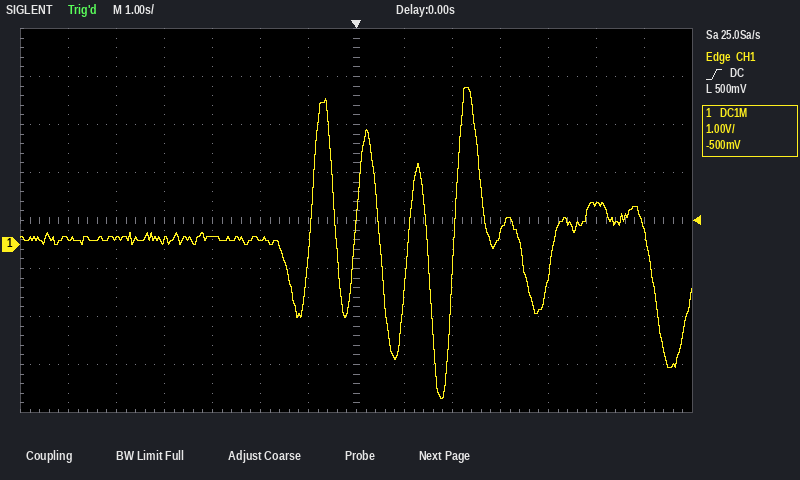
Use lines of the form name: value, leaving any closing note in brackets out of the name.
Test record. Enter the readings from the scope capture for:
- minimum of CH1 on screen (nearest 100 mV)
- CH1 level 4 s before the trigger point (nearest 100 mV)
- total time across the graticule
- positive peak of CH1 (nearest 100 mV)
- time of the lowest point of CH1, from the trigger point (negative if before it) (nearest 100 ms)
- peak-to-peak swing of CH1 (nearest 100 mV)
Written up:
minimum of CH1 on screen: -3.2 V
CH1 level 4 s before the trigger point: 100 mV
total time across the graticule: 14 s
positive peak of CH1: 3.3 V
time of the lowest point of CH1, from the trigger point (negative if before it): +1.8 s
peak-to-peak swing of CH1: 6.5 V
